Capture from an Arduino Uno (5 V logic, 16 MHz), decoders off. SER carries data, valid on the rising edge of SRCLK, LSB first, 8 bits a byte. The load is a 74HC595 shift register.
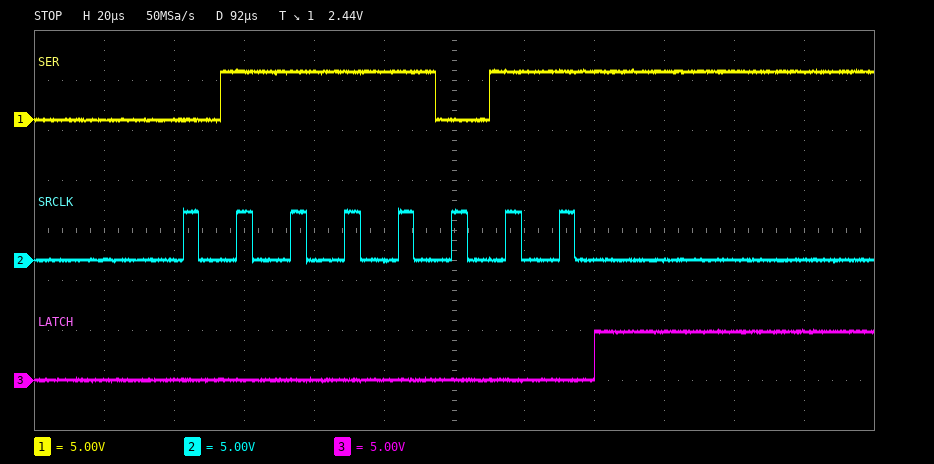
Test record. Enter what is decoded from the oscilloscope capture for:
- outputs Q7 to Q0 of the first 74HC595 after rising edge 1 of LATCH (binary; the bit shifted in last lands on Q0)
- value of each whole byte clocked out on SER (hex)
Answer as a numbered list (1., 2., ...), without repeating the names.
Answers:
1. 01111011
2. 0xDE
